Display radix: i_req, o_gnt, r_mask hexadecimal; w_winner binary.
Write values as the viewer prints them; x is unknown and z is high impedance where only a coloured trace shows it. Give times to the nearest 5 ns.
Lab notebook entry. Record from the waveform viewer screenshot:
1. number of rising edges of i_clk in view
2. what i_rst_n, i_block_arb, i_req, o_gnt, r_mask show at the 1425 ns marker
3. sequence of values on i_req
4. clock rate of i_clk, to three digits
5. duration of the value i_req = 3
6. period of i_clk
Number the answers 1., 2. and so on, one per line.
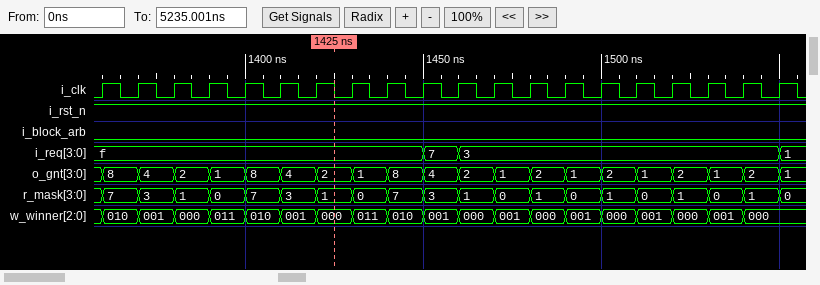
1. 20
2. i_rst_n=1, i_block_arb=0, i_req=f, o_gnt=2, r_mask=1
3. f, 7, 3, 1
4. 100 MHz
5. 90 ns
6. 10 ns
